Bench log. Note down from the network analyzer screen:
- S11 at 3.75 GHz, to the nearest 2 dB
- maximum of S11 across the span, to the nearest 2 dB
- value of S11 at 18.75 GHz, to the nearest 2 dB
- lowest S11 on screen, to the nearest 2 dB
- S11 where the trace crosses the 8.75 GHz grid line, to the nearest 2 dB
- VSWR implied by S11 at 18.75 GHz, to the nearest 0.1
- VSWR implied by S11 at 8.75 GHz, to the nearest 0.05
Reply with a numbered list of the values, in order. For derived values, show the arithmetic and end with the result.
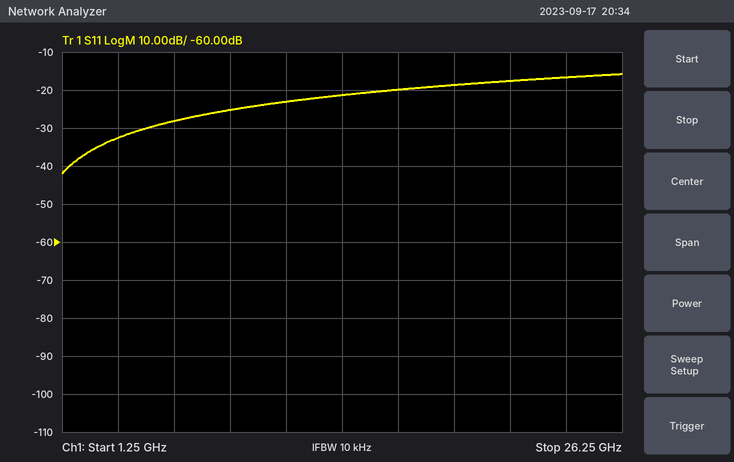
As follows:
1. -32 dB
2. -16 dB
3. -18 dB
4. -42 dB
5. -26 dB
6. |Γ| = 10^(-18/20) = 0.1259; VSWR = (1 + 0.1259)/(1 − 0.1259) ≈ 1.3
7. |Γ| = 10^(-26/20) = 0.0501; VSWR = (1 + 0.0501)/(1 − 0.0501) ≈ 1.11, so 1.10 to the nearest 0.05
